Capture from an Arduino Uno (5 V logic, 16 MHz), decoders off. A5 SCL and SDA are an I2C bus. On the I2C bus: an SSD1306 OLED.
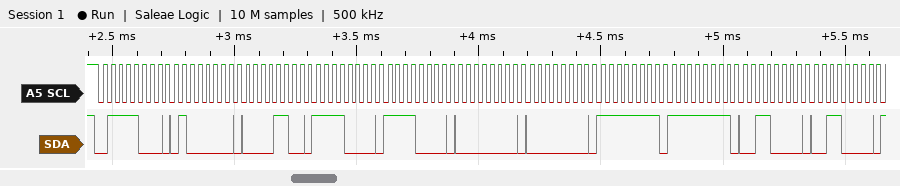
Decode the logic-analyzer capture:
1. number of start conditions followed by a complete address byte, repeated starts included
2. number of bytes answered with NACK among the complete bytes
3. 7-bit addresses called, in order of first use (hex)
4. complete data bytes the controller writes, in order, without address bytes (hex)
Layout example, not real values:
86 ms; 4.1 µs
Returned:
1; 0; 0x3C; 40 0C F0 F0 00 00 FF FF 30 30
